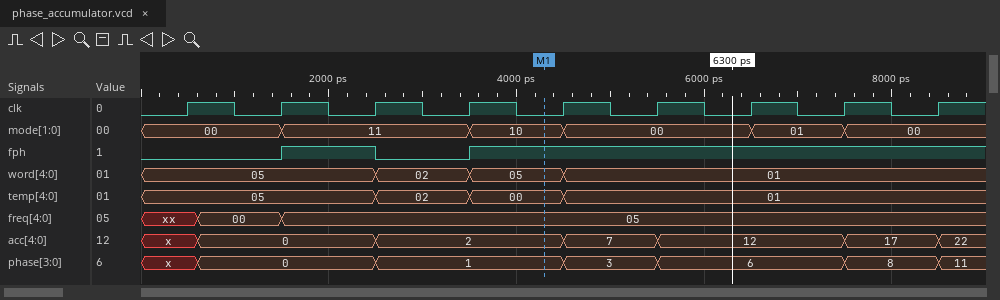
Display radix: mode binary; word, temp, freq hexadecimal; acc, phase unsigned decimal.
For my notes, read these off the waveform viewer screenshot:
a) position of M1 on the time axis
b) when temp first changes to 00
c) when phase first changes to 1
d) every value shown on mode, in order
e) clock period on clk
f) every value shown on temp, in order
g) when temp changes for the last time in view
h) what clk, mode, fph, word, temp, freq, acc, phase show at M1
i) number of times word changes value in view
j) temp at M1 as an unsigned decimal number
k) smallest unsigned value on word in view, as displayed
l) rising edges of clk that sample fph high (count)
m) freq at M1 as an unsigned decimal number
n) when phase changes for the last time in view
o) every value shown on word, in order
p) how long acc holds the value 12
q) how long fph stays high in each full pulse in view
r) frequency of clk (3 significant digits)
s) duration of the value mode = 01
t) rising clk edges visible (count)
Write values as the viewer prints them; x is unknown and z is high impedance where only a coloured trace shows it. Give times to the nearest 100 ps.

4300 ps
3500 ps
2500 ps
00, 11, 10, 00, 01, 00
1000 ps
05, 02, 00, 01
4500 ps
clk=0, mode=10, fph=1, word=05, temp=00, freq=05, acc=2, phase=1
3
0
01
6
5
8500 ps
05, 02, 05, 01
2000 ps
1000 ps
1.00 GHz
1000 ps
9
